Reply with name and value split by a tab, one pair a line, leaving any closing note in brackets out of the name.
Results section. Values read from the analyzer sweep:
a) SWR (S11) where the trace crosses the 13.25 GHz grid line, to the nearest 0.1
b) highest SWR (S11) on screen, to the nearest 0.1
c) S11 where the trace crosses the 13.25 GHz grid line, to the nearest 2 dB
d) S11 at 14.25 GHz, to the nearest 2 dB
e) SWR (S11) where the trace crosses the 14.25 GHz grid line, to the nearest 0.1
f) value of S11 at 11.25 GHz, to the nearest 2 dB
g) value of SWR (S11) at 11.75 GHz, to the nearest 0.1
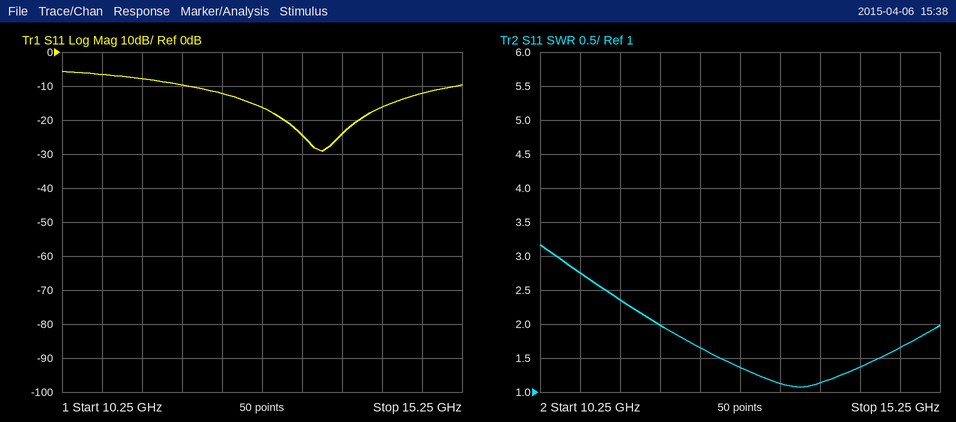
SWR (S11) where the trace crosses the 13.25 GHz grid line, to the nearest 0.1	1.1
highest SWR (S11) on screen, to the nearest 0.1	3.2
S11 where the trace crosses the 13.25 GHz grid line, to the nearest 2 dB	-24 dB
S11 at 14.25 GHz, to the nearest 2 dB	-16 dB
SWR (S11) where the trace crosses the 14.25 GHz grid line, to the nearest 0.1	1.4
value of S11 at 11.25 GHz, to the nearest 2 dB	-8 dB
value of SWR (S11) at 11.75 GHz, to the nearest 0.1	2.0
